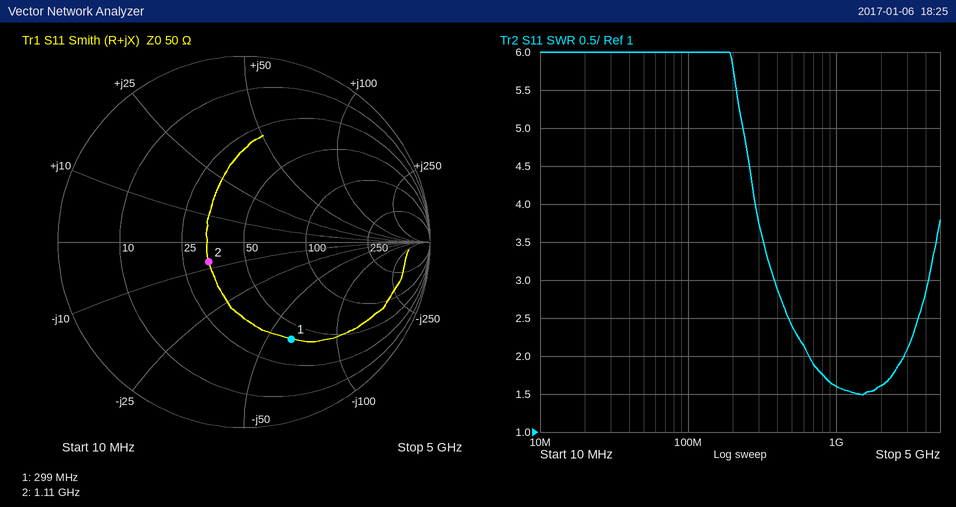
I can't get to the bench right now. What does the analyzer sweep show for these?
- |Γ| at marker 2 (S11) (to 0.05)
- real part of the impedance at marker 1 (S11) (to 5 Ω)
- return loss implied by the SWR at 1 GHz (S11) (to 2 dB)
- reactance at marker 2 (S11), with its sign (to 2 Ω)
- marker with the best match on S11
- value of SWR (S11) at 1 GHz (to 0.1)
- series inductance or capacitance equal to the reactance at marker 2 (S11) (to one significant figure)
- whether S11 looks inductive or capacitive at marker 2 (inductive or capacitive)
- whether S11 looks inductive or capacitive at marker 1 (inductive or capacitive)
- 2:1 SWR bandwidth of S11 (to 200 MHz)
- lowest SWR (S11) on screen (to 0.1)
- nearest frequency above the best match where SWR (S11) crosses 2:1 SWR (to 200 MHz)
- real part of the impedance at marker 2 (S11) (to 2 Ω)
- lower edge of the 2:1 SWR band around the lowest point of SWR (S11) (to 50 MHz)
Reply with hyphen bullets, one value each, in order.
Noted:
- 0.20
- 40 Ω
- 12 dB
- -8 Ω
- marker 2
- 1.6
- 20 pF
- capacitive
- capacitive
- 2.2 GHz
- 1.5
- 2.8 GHz
- 34 Ω
- 650 MHz
